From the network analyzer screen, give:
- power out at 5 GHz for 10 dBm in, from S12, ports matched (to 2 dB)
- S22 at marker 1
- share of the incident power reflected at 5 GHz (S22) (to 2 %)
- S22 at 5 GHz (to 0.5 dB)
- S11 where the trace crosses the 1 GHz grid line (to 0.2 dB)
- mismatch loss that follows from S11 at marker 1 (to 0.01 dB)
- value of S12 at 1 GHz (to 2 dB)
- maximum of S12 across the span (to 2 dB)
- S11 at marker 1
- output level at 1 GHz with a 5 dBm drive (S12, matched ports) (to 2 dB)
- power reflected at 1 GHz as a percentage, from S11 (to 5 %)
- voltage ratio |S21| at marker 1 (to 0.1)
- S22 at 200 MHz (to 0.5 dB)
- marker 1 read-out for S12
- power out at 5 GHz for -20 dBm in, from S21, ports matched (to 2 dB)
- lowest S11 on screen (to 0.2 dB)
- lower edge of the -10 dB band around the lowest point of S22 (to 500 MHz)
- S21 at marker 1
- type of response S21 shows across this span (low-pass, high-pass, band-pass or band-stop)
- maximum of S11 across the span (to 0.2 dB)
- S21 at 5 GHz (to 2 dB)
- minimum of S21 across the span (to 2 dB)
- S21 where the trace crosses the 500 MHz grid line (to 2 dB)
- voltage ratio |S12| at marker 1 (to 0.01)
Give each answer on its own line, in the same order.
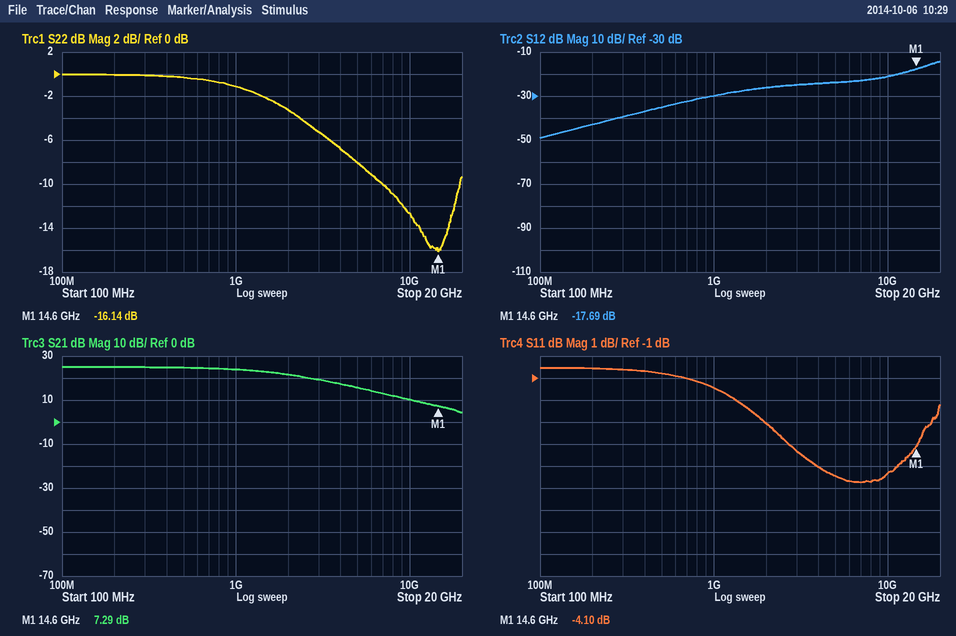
-14 dBm
-16.14 dB
16 %
-8.0 dB
-1.4 dB
2.14 dB
-30 dB
-14 dB
-4.10 dB
-24 dBm
70 %
2.3
0.0 dB
-17.69 dB
-4 dBm
-5.8 dB
7.0 GHz
7.29 dB
low-pass
-0.6 dB
16 dB
4 dB
24 dB
0.13
